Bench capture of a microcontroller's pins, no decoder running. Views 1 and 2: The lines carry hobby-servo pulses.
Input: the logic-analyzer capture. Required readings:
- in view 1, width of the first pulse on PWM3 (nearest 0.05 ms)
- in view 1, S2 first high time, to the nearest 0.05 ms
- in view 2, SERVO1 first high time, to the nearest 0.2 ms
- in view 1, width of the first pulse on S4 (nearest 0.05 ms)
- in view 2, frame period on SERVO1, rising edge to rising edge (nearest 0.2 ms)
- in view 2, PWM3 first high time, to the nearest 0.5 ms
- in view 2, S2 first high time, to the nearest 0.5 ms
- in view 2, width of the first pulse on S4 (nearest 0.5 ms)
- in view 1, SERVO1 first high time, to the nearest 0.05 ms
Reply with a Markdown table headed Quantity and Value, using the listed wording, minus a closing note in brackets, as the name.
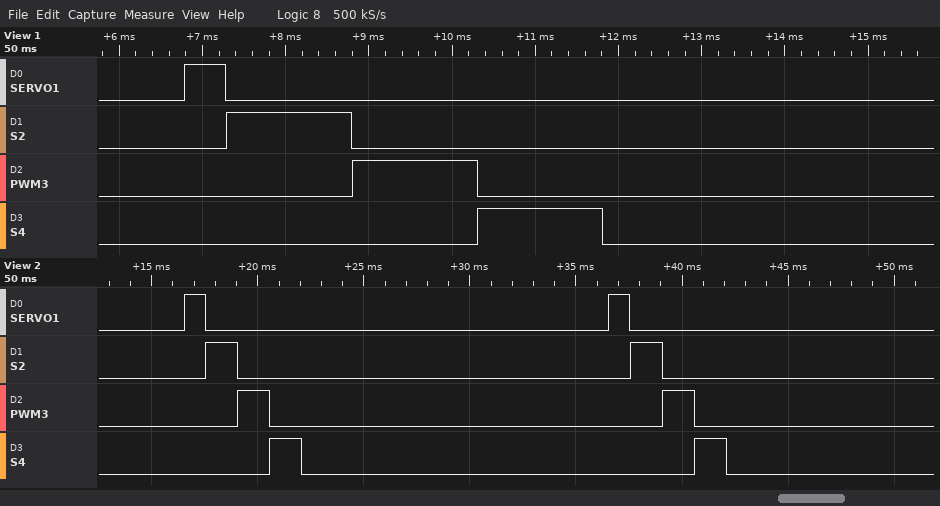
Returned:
| Quantity | Value |
|---|---|
| in view 1, width of the first pulse on PWM3 | 1.50 ms |
| in view 1, S2 first high time, to the nearest 0.05 ms | 1.50 ms |
| in view 2, SERVO1 first high time, to the nearest 0.2 ms | 1.0 ms |
| in view 1, width of the first pulse on S4 | 1.50 ms |
| in view 2, frame period on SERVO1, rising edge to rising edge | 20.0 ms |
| in view 2, PWM3 first high time, to the nearest 0.5 ms | 1.5 ms |
| in view 2, S2 first high time, to the nearest 0.5 ms | 1.5 ms |
| in view 2, width of the first pulse on S4 | 1.5 ms |
| in view 1, SERVO1 first high time, to the nearest 0.05 ms | 0.50 ms |
